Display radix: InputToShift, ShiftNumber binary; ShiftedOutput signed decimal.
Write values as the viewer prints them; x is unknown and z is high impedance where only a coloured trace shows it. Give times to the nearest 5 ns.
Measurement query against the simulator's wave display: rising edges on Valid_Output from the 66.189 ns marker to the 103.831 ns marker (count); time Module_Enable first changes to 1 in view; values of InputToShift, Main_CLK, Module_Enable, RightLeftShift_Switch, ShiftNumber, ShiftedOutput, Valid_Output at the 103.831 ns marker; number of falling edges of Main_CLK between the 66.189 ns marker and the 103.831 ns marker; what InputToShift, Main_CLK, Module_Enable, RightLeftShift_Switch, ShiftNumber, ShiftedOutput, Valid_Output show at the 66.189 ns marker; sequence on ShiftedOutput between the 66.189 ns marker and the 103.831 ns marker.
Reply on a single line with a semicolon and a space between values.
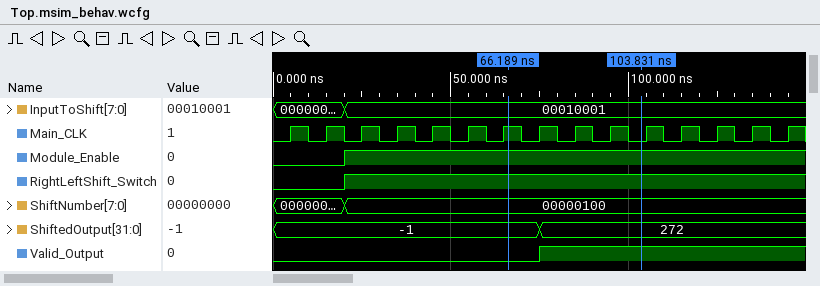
1; 20 ns; InputToShift=00010001, Main_CLK=0, Module_Enable=1, RightLeftShift_Switch=1, ShiftNumber=00000100, ShiftedOutput=272, Valid_Output=1; 4; InputToShift=00010001, Main_CLK=1, Module_Enable=1, RightLeftShift_Switch=1, ShiftNumber=00000100, ShiftedOutput=-1, Valid_Output=0; -1, 272
